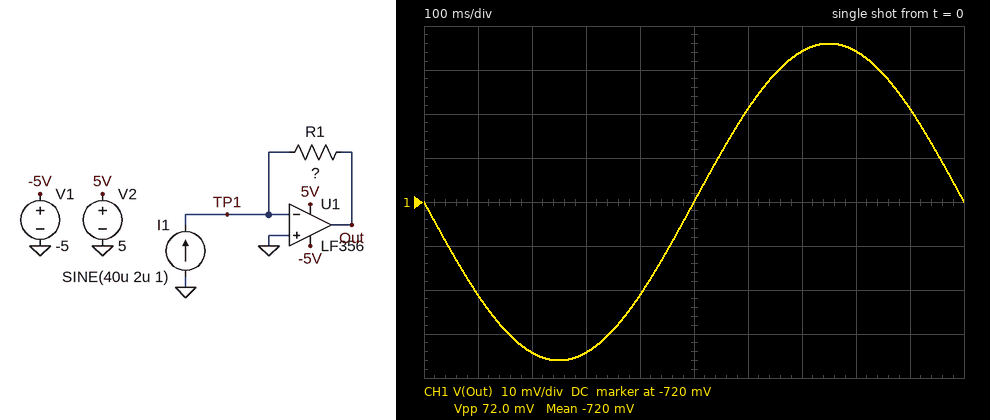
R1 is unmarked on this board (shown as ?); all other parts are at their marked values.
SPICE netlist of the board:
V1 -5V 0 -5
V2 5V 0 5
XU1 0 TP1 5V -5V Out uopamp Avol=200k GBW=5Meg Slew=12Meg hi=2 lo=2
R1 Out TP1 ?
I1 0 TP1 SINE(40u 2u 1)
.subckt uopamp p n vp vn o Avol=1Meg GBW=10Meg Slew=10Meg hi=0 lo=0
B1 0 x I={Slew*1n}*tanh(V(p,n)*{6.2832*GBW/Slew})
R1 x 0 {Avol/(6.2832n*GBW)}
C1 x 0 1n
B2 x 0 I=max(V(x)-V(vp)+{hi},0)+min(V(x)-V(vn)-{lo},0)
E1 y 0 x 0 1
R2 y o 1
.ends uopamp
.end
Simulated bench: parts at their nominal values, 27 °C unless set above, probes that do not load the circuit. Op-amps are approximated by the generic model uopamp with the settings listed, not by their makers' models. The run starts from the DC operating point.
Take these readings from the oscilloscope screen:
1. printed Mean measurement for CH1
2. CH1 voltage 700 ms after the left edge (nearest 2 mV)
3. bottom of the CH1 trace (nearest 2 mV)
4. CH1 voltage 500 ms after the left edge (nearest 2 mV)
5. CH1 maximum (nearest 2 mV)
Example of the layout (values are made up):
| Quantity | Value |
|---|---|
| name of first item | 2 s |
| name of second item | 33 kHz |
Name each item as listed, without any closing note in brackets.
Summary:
| Quantity | Value |
|---|---|
| printed Mean measurement for CH1 | -720 mV |
| CH1 voltage 700 ms after the left edge | -686 mV |
| bottom of the CH1 trace | -756 mV |
| CH1 voltage 500 ms after the left edge | -720 mV |
| CH1 maximum | -684 mV |
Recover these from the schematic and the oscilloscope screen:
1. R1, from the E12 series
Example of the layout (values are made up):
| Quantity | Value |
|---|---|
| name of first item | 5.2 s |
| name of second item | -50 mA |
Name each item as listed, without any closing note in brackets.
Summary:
| Quantity | Value |
|---|---|
| R1, from the E12 series | 18 kΩ |
